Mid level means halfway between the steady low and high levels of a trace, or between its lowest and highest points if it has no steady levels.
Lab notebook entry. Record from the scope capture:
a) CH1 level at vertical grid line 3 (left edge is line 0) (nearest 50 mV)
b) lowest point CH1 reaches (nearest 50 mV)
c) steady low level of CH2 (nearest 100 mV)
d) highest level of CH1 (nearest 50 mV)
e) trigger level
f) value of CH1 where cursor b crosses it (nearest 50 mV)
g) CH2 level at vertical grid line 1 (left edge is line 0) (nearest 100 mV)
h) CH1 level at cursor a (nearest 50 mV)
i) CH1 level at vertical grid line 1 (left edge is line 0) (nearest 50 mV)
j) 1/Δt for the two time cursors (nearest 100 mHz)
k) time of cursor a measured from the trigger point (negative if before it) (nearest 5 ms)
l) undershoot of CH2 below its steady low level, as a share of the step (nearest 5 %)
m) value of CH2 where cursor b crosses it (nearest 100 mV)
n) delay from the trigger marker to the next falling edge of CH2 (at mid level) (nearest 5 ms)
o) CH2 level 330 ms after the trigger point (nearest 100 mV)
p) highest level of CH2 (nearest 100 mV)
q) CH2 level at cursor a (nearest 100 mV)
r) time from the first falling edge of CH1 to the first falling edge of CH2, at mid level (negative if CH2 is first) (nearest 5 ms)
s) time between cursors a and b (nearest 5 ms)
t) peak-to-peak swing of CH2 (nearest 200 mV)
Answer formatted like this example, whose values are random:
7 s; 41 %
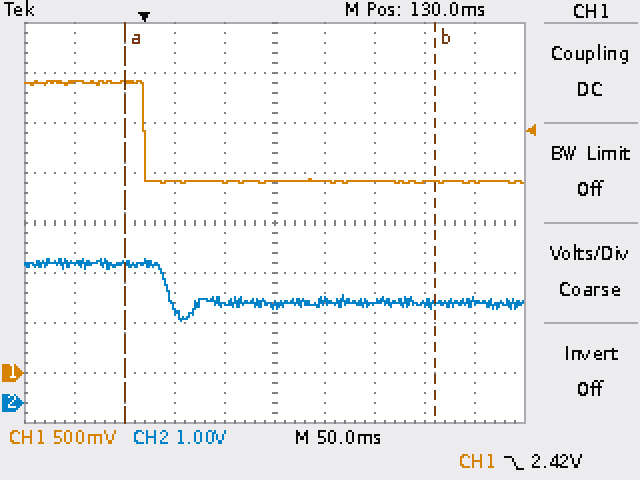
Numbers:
1.90 V; 1.90 V; 2.0 V; 2.90 V; 2.42 V; 1.90 V; 2.8 V; 2.90 V; 2.90 V; 3.2 Hz; -20 ms; 45 %; 2.0 V; 20 ms; 2.0 V; 2.9 V; 2.8 V; +20 ms; 310 ms; 1.2 V
